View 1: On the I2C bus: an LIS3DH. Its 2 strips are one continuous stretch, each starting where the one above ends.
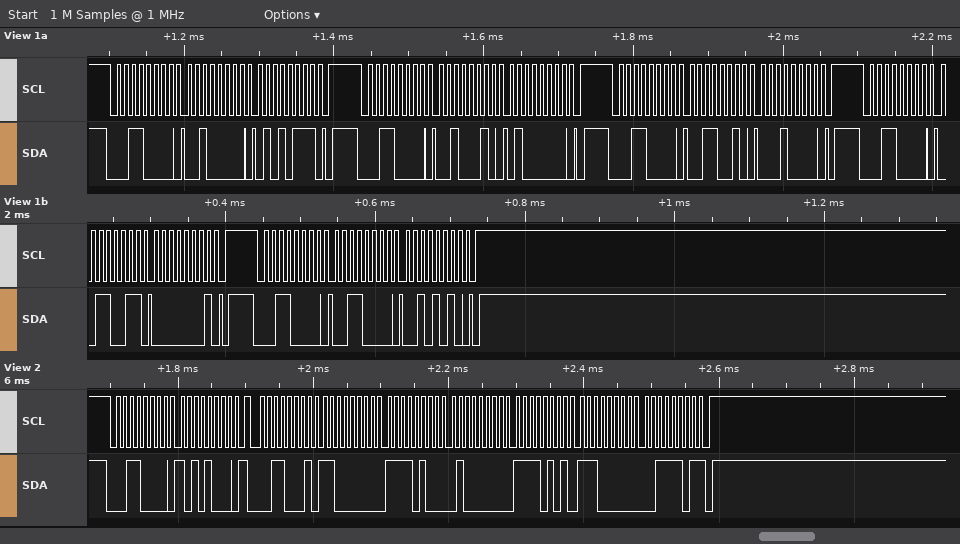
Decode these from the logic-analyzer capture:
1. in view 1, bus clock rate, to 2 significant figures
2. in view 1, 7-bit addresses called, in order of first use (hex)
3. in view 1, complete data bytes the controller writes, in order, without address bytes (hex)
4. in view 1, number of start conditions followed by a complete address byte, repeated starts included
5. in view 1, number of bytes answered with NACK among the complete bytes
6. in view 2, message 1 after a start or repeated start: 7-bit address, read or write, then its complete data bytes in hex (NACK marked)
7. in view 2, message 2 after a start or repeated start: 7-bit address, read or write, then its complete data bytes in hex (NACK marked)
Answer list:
100 kHz
0x18
20 57 22 40 32 10 33 01 30 2A
5
0
0x18 write: A8
0x18 read: C0 F4 40 F5 E0 3D NACK
